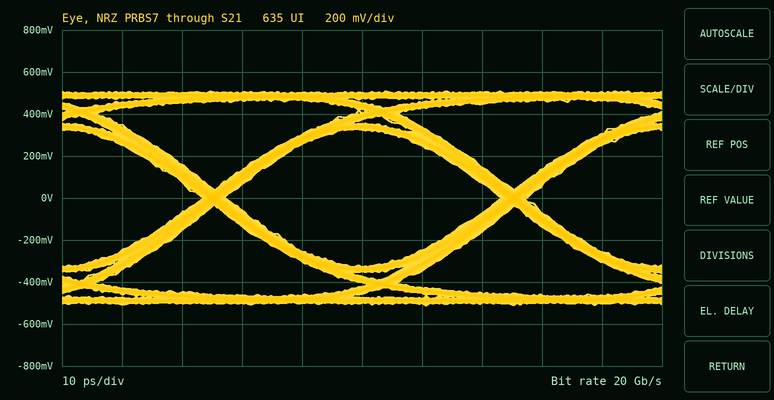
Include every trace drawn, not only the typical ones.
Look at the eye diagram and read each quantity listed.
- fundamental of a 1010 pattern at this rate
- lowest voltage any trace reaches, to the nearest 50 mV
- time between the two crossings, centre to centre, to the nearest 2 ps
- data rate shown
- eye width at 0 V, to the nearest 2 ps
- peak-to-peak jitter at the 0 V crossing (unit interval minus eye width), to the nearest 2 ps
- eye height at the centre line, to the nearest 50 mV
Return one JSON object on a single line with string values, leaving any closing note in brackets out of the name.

{"fundamental of a 1010 pattern at this rate": "10 GHz", "lowest voltage any trace reaches, to the nearest 50 mV": "-500 mV", "time between the two crossings, centre to centre, to the nearest 2 ps": "50 ps", "data rate shown": "20 Gb/s", "eye width at 0 V, to the nearest 2 ps": "46 ps", "peak-to-peak jitter at the 0 V crossing (unit interval minus eye width), to the nearest 2 ps": "4 ps", "eye height at the centre line, to the nearest 50 mV": "650 mV"}
